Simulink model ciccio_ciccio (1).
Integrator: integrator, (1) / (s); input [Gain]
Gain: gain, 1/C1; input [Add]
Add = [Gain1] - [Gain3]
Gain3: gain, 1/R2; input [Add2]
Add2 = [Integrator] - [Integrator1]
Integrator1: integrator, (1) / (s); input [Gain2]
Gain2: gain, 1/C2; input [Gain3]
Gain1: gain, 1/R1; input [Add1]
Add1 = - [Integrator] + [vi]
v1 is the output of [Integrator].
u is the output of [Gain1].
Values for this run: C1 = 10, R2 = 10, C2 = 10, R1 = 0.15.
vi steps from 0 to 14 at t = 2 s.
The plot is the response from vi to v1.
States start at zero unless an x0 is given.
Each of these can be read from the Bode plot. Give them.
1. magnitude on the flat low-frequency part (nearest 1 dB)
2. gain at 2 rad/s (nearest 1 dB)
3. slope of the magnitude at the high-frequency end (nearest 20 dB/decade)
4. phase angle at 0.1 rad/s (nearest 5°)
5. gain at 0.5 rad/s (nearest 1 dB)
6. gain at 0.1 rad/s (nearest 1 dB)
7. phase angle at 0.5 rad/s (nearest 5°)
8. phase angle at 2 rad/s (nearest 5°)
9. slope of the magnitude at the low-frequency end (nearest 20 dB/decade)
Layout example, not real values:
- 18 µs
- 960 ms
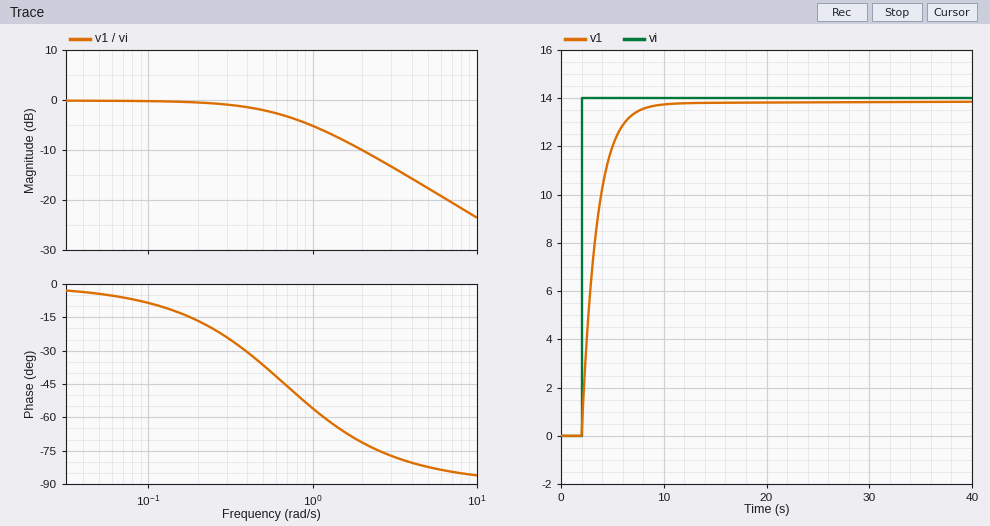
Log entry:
- 0 dB
- -10 dB
- -20 dB/decade
- -10°
- -2 dB
- 0 dB
- -35°
- -70°
- 0 dB/decade
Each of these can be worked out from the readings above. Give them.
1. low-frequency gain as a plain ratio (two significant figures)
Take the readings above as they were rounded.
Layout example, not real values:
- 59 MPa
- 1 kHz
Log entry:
- 1.0
